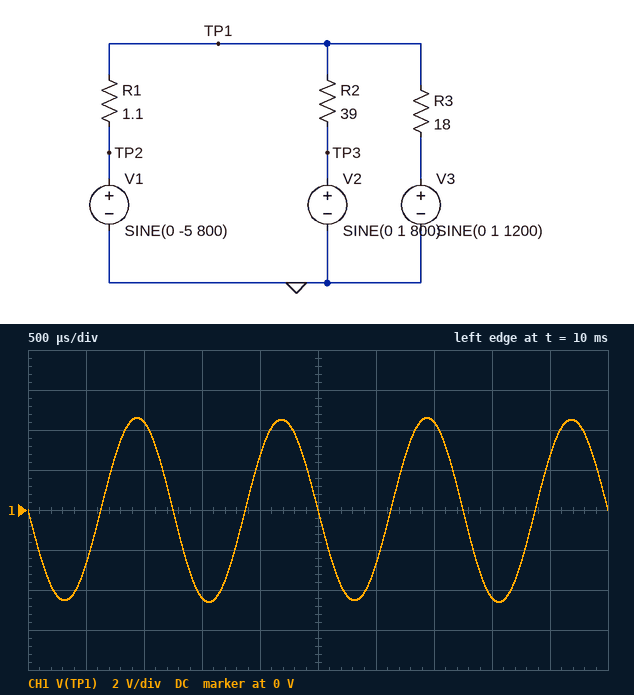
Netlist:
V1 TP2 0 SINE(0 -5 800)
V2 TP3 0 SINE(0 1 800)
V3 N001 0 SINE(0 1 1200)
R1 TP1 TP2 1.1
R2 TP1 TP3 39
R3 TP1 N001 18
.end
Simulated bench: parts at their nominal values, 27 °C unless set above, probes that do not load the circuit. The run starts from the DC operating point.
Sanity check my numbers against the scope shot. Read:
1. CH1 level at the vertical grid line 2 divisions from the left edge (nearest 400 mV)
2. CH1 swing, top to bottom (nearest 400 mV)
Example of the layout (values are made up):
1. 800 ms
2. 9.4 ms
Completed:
1. 4.4 V
2. 9.2 V
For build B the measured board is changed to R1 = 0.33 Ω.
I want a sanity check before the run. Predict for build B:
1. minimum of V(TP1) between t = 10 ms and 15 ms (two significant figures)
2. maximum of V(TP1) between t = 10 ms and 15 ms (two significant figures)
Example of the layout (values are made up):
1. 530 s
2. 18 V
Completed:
1. -4.9 V
2. 4.9 V
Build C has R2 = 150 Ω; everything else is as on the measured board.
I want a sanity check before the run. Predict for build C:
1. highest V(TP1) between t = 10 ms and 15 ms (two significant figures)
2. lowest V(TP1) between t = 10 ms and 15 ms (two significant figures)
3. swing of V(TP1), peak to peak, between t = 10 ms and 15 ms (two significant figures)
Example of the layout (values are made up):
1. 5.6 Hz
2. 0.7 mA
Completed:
1. 4.7 V
2. -4.7 V
3. 9.4 V
